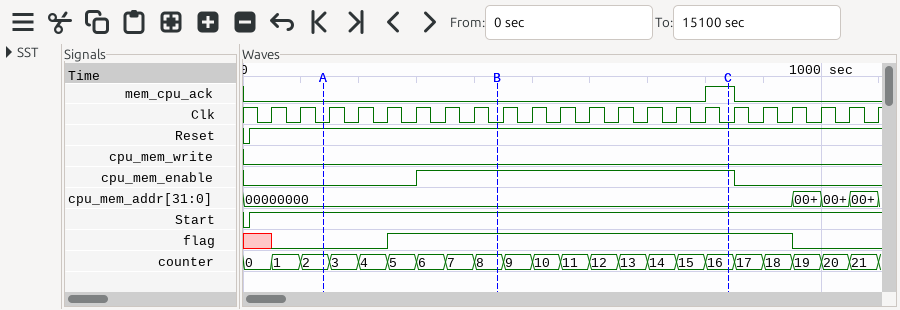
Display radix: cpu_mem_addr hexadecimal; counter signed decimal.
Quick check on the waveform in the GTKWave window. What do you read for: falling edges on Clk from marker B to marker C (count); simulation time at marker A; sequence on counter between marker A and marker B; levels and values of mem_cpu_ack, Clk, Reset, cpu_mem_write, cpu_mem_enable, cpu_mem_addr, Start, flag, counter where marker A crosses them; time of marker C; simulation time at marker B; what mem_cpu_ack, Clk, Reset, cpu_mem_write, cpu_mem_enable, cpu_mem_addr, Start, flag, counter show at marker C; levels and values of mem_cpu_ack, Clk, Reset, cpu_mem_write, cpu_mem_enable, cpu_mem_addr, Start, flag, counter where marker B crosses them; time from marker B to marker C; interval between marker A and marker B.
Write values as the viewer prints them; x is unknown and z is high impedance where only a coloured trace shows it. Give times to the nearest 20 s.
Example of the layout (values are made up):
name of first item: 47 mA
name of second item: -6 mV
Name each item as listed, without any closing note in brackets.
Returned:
falling edges on Clk from marker B to marker C: 8
simulation time at marker A: 140 s
sequence on counter between marker A and marker B: 2, 3, 4, 5, 6, 7, 8
levels and values of mem_cpu_ack, Clk, Reset, cpu_mem_write, cpu_mem_enable, cpu_mem_addr, Start, flag, counter where marker A crosses them: mem_cpu_ack=0, Clk=0, Reset=1, cpu_mem_write=0, cpu_mem_enable=0, cpu_mem_addr=00000000, Start=1, flag=0, counter=2
time of marker C: 840 s
simulation time at marker B: 440 s
what mem_cpu_ack, Clk, Reset, cpu_mem_write, cpu_mem_enable, cpu_mem_addr, Start, flag, counter show at marker C: mem_cpu_ack=1, Clk=0, Reset=1, cpu_mem_write=0, cpu_mem_enable=1, cpu_mem_addr=00000000, Start=1, flag=1, counter=16
levels and values of mem_cpu_ack, Clk, Reset, cpu_mem_write, cpu_mem_enable, cpu_mem_addr, Start, flag, counter where marker B crosses them: mem_cpu_ack=0, Clk=0, Reset=1, cpu_mem_write=0, cpu_mem_enable=1, cpu_mem_addr=00000000, Start=1, flag=1, counter=8
time from marker B to marker C: 400 s
interval between marker A and marker B: 300 s
